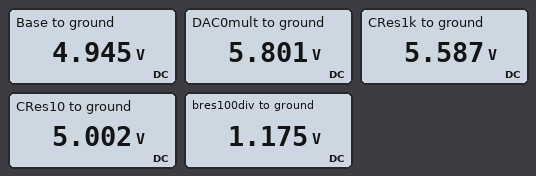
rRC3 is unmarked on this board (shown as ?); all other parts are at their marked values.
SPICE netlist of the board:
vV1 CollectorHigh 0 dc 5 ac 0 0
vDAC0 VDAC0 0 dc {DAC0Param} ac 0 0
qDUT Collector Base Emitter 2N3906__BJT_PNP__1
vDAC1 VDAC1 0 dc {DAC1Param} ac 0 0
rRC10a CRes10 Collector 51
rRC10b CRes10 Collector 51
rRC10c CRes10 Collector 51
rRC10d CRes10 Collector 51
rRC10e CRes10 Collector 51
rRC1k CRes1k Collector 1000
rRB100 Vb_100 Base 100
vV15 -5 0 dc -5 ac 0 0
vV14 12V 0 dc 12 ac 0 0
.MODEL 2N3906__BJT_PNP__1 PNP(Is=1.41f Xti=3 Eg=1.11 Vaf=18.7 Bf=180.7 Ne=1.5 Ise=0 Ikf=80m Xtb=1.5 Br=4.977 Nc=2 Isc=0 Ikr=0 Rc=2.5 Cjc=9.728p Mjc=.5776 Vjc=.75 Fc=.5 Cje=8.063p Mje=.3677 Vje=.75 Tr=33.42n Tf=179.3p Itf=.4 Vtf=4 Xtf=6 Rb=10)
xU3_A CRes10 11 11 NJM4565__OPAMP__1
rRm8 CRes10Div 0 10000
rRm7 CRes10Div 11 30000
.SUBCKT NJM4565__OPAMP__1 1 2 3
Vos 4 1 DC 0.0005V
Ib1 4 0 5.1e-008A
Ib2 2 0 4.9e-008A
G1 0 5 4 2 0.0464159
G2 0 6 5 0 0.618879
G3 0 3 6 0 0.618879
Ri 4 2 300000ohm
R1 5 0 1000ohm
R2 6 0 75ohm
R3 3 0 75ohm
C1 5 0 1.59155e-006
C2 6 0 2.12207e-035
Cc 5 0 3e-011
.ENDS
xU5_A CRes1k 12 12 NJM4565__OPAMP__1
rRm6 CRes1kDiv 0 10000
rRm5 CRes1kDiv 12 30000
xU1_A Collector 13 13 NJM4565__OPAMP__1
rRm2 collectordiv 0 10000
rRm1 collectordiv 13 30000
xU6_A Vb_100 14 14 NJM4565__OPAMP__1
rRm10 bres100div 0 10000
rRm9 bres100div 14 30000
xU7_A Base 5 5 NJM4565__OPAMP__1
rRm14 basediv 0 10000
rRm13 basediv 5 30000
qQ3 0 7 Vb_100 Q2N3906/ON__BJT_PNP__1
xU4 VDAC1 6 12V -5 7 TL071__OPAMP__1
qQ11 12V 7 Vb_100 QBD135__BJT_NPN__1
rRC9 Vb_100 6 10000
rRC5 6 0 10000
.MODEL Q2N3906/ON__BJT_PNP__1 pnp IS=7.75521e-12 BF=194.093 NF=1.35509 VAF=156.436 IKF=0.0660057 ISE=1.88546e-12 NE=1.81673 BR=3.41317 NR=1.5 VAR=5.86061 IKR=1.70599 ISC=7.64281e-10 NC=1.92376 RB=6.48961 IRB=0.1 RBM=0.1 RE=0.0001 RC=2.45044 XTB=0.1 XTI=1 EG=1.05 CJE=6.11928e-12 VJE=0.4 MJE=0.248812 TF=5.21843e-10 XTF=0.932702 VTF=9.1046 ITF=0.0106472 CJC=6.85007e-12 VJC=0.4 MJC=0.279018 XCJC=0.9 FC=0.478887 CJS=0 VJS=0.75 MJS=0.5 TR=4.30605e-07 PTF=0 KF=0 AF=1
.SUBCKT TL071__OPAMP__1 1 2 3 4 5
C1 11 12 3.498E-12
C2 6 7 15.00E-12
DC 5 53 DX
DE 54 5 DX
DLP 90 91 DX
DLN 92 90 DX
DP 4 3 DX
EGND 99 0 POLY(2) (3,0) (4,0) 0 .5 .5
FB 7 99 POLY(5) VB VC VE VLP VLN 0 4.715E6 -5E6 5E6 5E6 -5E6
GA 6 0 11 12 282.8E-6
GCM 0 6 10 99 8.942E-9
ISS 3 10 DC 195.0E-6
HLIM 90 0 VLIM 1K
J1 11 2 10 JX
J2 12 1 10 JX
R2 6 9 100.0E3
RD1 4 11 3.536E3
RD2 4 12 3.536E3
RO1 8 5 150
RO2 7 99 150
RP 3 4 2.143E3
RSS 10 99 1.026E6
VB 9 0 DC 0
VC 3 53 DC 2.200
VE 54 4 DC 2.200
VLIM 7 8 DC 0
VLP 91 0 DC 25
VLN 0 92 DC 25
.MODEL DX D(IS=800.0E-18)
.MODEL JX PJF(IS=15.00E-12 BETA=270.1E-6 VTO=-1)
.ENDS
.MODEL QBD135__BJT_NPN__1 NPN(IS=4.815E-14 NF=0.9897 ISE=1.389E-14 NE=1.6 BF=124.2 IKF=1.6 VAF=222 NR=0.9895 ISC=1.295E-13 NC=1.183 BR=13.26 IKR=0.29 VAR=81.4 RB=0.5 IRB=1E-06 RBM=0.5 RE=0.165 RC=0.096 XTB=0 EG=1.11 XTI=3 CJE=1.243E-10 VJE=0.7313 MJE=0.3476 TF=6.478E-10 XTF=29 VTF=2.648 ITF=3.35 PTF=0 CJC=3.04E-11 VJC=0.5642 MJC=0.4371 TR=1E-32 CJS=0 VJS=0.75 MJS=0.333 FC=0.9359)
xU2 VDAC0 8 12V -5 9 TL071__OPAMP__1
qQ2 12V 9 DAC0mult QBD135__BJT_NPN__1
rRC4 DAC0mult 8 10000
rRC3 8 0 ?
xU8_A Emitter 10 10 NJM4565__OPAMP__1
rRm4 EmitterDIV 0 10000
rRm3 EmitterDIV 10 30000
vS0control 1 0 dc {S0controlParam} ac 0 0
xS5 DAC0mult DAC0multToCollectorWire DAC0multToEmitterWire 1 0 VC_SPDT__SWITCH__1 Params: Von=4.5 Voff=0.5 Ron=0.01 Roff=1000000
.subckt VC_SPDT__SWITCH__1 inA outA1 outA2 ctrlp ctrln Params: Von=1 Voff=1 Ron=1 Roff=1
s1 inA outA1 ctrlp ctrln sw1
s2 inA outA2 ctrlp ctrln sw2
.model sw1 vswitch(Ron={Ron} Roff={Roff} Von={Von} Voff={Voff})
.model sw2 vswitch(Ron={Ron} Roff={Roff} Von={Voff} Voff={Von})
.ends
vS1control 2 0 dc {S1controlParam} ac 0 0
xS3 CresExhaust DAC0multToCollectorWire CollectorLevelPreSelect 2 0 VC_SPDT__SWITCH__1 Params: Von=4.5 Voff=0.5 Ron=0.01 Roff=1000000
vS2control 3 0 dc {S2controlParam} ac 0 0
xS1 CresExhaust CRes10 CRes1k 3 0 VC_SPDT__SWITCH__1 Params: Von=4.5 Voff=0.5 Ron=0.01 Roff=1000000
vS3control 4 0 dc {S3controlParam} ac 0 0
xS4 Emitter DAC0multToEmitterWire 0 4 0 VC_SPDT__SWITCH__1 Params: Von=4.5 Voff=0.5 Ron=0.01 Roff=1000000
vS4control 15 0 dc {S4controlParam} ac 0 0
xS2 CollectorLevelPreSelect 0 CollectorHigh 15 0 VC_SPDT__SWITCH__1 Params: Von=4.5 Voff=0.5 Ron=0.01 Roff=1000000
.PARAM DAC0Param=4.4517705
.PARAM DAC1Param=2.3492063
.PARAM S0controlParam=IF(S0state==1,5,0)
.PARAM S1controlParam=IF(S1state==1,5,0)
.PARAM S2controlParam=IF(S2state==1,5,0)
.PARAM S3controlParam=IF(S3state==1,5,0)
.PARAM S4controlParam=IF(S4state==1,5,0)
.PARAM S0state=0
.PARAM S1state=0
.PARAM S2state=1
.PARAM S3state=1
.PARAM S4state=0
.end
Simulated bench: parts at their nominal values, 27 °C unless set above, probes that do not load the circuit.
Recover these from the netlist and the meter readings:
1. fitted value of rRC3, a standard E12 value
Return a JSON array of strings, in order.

["33 kΩ"]
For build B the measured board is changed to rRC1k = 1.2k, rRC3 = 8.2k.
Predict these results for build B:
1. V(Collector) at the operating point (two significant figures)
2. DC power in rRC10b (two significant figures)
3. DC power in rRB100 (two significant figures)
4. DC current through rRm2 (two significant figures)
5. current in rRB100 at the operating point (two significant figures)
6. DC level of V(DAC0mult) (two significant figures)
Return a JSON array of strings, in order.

["8.6 V", "260 mW", "130 mW", "220 µA", "36 mA", "9.6 V"]
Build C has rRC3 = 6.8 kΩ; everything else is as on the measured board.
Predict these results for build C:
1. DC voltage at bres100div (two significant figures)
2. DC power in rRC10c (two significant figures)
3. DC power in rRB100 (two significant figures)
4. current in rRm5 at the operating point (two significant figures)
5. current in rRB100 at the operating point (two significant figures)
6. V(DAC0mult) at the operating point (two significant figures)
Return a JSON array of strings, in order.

["1.2 V", "260 mW", "130 mW", "220 µA", "37 mA", "9.6 V"]
